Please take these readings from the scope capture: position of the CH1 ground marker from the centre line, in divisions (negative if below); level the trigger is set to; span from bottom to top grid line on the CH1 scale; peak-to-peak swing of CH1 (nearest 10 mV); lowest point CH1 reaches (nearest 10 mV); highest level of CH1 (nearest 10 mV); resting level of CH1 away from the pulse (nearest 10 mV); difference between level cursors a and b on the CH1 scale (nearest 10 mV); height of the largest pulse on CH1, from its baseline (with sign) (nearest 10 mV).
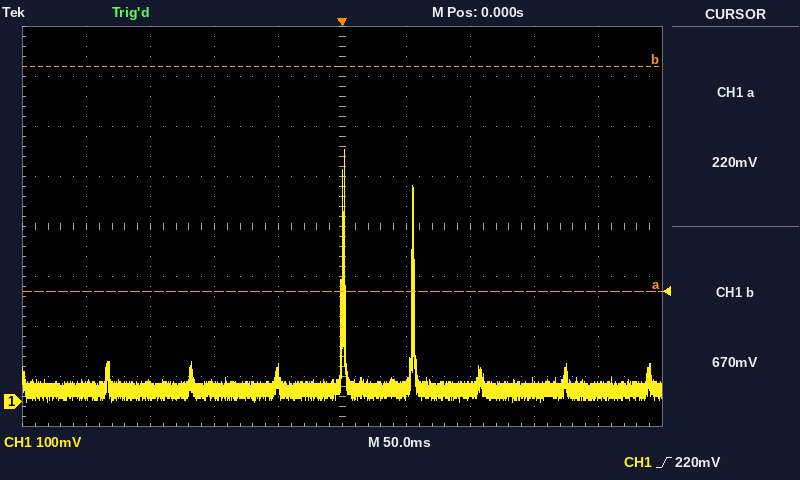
-3.5 div
220 mV
800 mV
500 mV
0 mV
500 mV
20 mV
450 mV
+480 mV
